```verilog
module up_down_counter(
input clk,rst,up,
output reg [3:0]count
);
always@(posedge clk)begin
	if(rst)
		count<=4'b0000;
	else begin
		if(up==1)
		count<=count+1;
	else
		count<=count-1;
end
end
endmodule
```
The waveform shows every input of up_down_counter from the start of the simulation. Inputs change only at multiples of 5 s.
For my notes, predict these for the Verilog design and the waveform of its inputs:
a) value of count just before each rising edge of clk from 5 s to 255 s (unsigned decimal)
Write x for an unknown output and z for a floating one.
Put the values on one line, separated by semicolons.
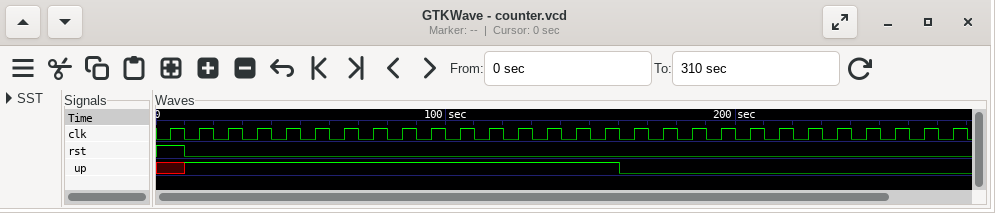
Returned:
x, 0, 1, 2, 3, 4, 5, 6, 7, 8, 9, 10, 11, 12, 13, 14, 15, 14, 13, 12, 11, 10, 9, 8, 7, 6
